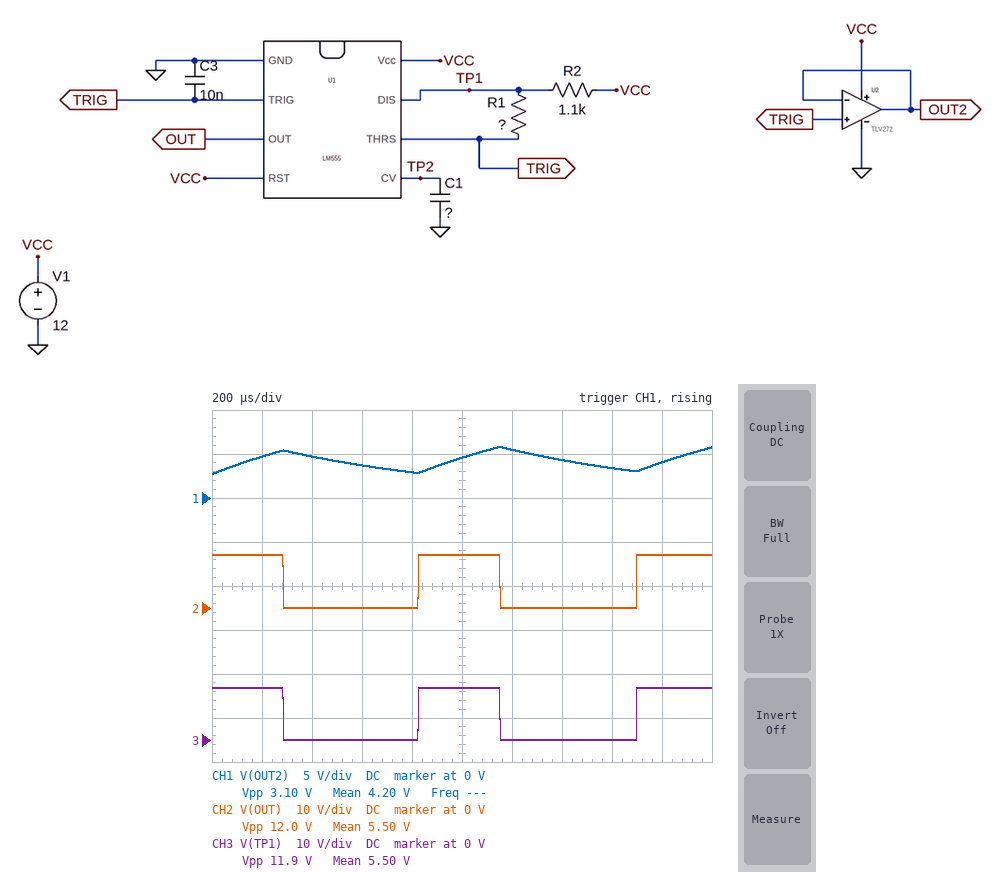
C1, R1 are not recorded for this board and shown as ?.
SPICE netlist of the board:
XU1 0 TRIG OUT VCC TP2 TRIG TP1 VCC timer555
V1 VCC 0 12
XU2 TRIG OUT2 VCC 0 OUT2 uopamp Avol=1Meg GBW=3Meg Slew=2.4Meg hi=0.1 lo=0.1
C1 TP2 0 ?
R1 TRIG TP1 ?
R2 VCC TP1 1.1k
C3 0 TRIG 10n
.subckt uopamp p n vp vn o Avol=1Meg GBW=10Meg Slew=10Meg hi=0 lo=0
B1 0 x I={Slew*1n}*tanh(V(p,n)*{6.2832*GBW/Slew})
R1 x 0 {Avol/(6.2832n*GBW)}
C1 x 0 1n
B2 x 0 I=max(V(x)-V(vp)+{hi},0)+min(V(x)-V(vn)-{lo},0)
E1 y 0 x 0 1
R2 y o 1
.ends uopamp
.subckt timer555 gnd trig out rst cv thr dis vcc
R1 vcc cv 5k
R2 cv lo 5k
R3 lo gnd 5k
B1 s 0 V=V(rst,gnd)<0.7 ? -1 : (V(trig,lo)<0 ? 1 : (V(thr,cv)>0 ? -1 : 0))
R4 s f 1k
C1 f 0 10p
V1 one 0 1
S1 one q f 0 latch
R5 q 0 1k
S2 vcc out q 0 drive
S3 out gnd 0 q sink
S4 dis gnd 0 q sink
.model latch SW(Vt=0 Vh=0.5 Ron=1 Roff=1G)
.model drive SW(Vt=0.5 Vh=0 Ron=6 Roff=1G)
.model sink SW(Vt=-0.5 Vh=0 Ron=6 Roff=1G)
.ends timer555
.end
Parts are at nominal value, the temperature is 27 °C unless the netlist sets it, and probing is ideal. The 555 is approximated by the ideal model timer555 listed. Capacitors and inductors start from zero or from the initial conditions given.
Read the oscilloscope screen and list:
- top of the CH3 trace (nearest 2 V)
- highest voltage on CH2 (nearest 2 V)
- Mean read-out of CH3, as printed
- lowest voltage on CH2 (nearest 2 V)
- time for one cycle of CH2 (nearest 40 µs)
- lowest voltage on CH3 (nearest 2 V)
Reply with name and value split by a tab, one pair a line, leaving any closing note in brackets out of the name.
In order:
top of the CH3 trace	12 V
highest voltage on CH2	12 V
Mean read-out of CH3, as printed	5.50 V
lowest voltage on CH2	0 V
time for one cycle of CH2	880 µs
lowest voltage on CH3	0 V
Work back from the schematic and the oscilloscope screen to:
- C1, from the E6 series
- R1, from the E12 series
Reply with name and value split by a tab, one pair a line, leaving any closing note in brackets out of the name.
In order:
C1, from the E6 series	1.5 µF
R1, from the E12 series	82 kΩ
